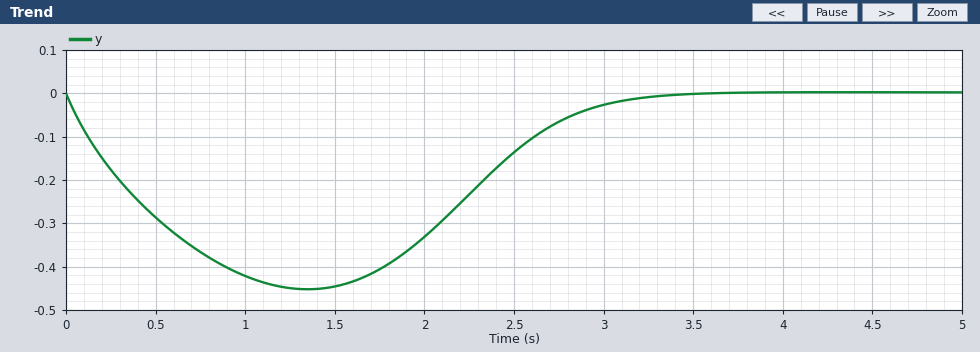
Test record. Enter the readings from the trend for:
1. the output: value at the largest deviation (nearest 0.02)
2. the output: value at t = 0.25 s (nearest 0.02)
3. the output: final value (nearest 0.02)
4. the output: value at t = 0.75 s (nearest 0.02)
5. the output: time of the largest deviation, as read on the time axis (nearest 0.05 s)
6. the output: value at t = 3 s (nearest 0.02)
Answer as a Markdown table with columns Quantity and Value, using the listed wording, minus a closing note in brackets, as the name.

| Quantity | Value |
|---|---|
| the output: value at the largest deviation | -0.46 |
| the output: value at t = 0.25 s | -0.18 |
| the output: final value | 0.00 |
| the output: value at t = 0.75 s | -0.36 |
| the output: time of the largest deviation, as read on the time axis | 1.35 s |
| the output: value at t = 3 s | -0.02 |
